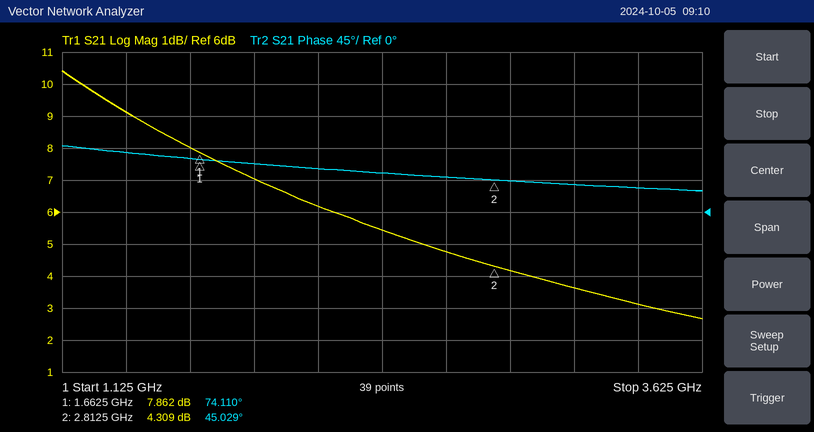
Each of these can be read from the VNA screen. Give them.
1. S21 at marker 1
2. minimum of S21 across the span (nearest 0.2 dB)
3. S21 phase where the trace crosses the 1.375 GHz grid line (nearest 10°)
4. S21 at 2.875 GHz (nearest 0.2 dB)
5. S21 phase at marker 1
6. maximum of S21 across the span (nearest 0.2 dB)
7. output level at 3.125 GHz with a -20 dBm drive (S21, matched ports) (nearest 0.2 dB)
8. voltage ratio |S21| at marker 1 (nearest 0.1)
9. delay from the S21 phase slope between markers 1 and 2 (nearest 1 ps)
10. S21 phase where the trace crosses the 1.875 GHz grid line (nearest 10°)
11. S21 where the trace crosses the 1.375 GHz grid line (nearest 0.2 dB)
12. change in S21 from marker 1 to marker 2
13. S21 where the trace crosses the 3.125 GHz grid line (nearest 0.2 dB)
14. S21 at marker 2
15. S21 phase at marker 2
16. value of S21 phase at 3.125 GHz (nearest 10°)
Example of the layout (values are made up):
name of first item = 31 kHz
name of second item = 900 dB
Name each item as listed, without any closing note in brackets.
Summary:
S21 at marker 1 = 7.862 dB
minimum of S21 across the span = 2.6 dB
S21 phase where the trace crosses the 1.375 GHz grid line = 80°
S21 at 2.875 GHz = 4.2 dB
S21 phase at marker 1 = 74.110°
maximum of S21 across the span = 10.4 dB
output level at 3.125 GHz with a -20 dBm drive (S21, matched ports) = -16.4 dBm
voltage ratio |S21| at marker 1 = 2.5
delay from the S21 phase slope between markers 1 and 2 = 70 ps
S21 phase where the trace crosses the 1.875 GHz grid line = 70°
S21 where the trace crosses the 1.375 GHz grid line = 9.2 dB
change in S21 from marker 1 to marker 2 = -3.553 dB
S21 where the trace crosses the 3.125 GHz grid line = 3.6 dB
S21 at marker 2 = 4.309 dB
S21 phase at marker 2 = 45.029°
value of S21 phase at 3.125 GHz = 40°
